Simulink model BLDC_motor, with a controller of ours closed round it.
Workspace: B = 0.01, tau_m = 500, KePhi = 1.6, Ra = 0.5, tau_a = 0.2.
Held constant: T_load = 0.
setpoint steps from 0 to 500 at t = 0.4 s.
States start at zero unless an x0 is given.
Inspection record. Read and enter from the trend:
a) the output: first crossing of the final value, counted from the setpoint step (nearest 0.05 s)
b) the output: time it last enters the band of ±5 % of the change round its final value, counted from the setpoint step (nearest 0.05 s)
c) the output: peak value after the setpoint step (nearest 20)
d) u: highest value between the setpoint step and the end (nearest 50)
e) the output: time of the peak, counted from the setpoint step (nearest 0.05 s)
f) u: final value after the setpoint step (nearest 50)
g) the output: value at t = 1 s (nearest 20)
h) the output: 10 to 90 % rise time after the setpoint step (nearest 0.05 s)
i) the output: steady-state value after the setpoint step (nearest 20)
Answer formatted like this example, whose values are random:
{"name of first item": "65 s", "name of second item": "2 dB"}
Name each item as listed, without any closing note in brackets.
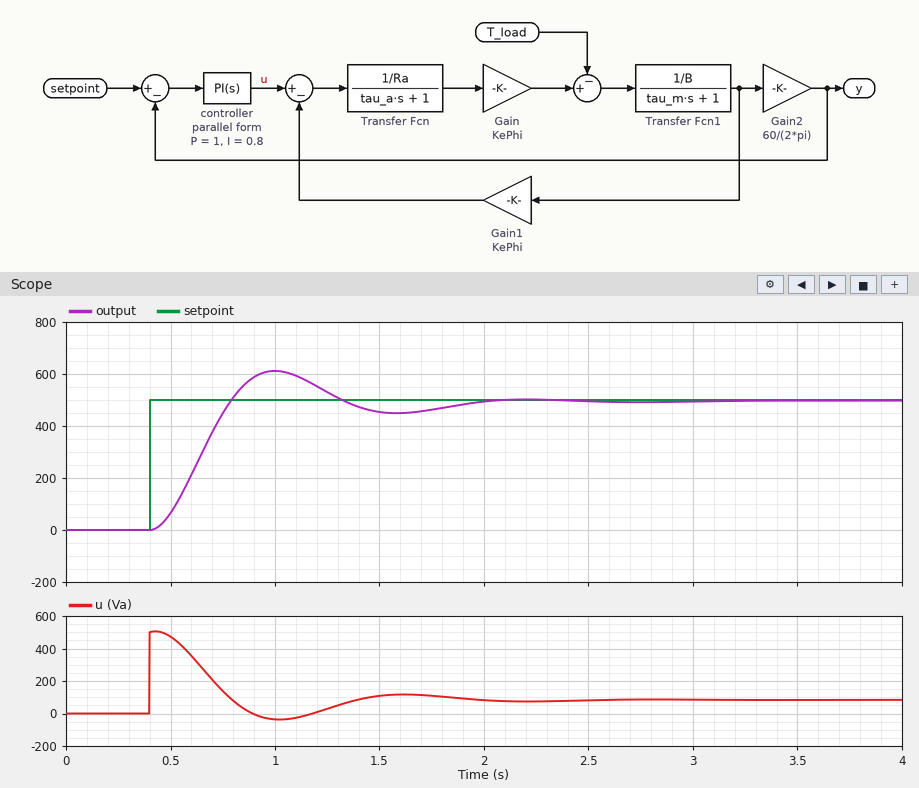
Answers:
{"the output: first crossing of the final value, counted from the setpoint step": "0.40 s", "the output: time it last enters the band of ±5 % of the change round its final value, counted from the setpoint step": "1.45 s", "the output: peak value after the setpoint step": "620", "u: highest value between the setpoint step and the end": "500", "the output: time of the peak, counted from the setpoint step": "0.60 s", "u: final value after the setpoint step": "100", "the output: value at t = 1 s": "620", "the output: 10 to 90 % rise time after the setpoint step": "0.25 s", "the output: steady-state value after the setpoint step": "500"}
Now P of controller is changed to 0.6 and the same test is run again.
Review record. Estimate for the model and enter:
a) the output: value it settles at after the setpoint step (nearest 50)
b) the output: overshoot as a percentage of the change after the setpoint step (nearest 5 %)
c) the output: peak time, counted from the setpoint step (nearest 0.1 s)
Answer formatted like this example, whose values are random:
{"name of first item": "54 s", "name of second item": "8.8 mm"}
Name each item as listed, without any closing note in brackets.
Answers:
{"the output: value it settles at after the setpoint step": "500", "the output: overshoot as a percentage of the change after the setpoint step": "20 %", "the output: peak time, counted from the setpoint step": "0.8 s"}
